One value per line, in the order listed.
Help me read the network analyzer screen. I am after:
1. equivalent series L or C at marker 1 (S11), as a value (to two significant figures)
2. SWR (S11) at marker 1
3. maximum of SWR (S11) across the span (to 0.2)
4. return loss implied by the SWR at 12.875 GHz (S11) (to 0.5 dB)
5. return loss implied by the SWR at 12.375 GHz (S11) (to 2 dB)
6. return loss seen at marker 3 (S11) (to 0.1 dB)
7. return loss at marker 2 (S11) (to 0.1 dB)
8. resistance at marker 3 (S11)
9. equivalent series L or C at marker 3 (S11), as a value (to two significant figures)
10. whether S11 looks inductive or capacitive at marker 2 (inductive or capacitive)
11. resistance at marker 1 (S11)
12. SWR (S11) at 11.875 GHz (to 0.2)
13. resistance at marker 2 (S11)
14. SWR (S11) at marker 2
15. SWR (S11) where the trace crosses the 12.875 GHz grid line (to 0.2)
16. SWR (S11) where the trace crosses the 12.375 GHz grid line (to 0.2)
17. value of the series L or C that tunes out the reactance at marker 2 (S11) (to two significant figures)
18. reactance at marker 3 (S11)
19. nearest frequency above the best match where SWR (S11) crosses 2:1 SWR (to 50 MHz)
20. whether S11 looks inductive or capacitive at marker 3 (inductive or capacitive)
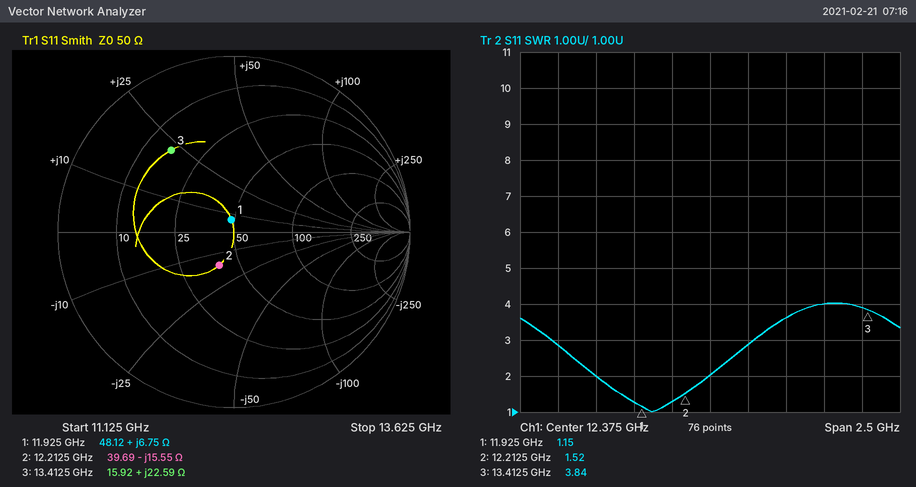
90 pH
1.15
4.0
5.0 dB
10 dB
4.6 dB
13.8 dB
15.92 Ω
270 pH
capacitive
48.12 Ω
1.2
39.69 Ω
1.52
3.6
2.0
200 pH
+22.59 Ω
12.35 GHz
inductive
